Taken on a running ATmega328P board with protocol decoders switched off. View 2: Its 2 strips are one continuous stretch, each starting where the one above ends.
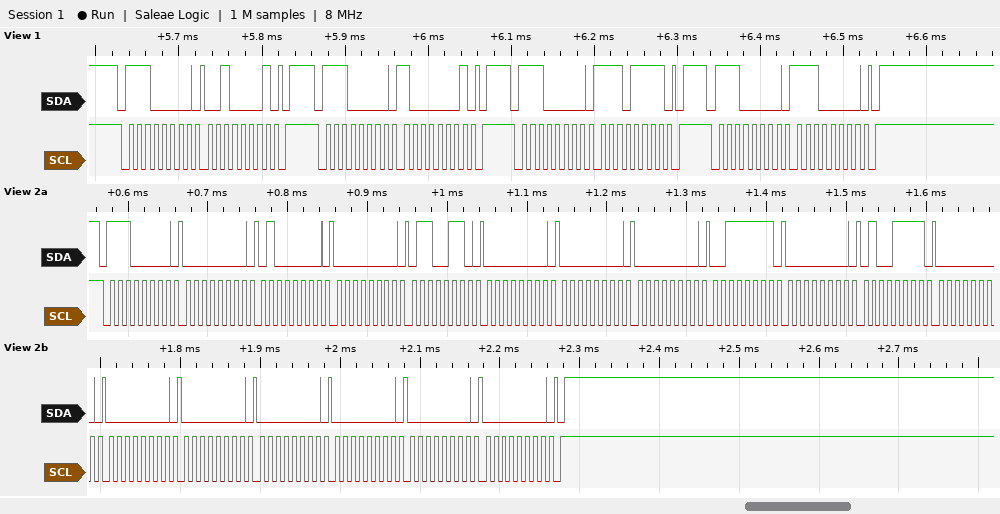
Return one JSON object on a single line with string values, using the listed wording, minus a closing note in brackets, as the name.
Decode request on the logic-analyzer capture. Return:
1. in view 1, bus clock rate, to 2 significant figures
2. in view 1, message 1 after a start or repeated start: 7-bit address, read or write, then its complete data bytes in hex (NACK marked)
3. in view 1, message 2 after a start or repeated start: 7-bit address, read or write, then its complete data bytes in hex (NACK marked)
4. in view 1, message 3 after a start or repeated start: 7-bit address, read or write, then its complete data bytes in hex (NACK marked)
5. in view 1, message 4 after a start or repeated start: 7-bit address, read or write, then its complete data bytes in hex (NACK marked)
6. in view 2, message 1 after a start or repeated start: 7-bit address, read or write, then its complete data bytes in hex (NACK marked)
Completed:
{"in view 1, bus clock rate, to 2 significant figures": "100 kHz", "in view 1, message 1 after a start or repeated start: 7-bit address, read or write, then its complete data bytes in hex": "0x70 write: 21", "in view 1, message 2 after a start or repeated start: 7-bit address, read or write, then its complete data bytes in hex": "0x70 write: 81", "in view 1, message 3 after a start or repeated start: 7-bit address, read or write, then its complete data bytes in hex": "0x70 write: EF", "in view 1, message 4 after a start or repeated start: 7-bit address, read or write, then its complete data bytes in hex": "0x70 write: E0", "in view 2, message 1 after a start or repeated start: 7-bit address, read or write, then its complete data bytes in hex": "0x70 write: 00 40 00 66 00 00 00 3F 00 4F 00 00 00 00 00 00 00"}
